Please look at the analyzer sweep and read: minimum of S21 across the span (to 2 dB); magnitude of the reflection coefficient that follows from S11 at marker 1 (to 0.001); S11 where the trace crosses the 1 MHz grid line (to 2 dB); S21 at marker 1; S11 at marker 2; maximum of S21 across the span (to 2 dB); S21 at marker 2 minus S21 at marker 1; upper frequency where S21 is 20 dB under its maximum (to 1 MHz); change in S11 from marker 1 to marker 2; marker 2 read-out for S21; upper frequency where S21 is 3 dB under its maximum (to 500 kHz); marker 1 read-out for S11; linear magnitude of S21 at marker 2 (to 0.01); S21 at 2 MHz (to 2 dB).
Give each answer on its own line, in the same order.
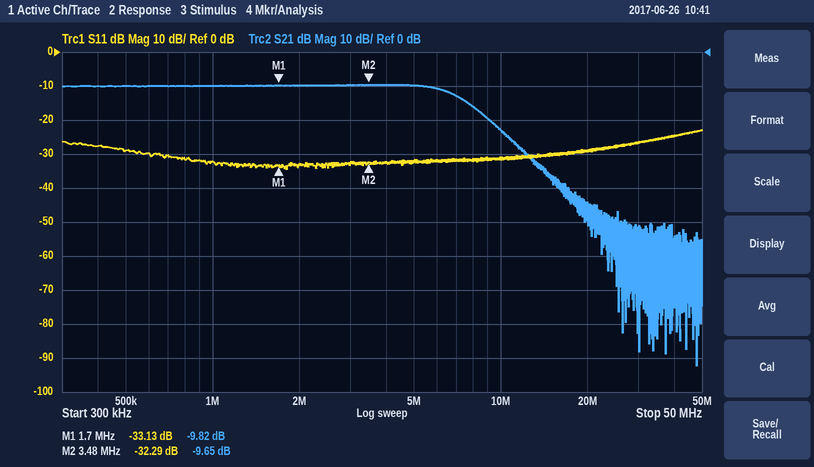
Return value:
-92 dB
0.022
-32 dB
-9.82 dB
-32.29 dB
-10 dB
0.17 dB
12 MHz
0.84 dB
-9.65 dB
7.0 MHz
-33.13 dB
0.33
-10 dB
